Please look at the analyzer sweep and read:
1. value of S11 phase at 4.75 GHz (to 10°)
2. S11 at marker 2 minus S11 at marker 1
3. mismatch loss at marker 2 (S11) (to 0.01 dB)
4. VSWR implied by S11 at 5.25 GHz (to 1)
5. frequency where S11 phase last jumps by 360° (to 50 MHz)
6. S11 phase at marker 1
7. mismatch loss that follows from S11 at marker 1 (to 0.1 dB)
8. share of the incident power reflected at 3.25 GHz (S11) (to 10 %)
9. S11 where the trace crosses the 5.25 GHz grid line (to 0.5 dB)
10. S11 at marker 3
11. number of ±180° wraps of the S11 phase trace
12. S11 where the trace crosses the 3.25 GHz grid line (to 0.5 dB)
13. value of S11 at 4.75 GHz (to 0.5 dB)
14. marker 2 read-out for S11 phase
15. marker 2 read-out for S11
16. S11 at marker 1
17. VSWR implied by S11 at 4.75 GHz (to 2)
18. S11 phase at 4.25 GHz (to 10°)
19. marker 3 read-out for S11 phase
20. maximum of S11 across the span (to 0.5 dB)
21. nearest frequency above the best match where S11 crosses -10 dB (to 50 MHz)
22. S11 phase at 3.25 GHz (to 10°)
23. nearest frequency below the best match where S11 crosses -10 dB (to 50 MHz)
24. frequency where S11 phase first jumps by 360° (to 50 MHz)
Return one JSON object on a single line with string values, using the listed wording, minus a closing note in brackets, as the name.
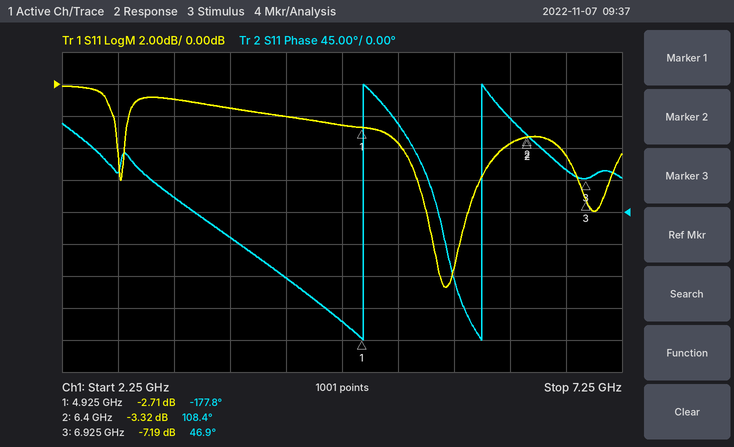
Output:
{"value of S11 phase at 4.75 GHz": "-150°", "S11 at marker 2 minus S11 at marker 1": "-0.61 dB", "mismatch loss at marker 2 (S11)": "2.72 dB", "VSWR implied by S11 at 5.25 GHz": "5", "frequency where S11 phase last jumps by 360°": "6.00 GHz", "S11 phase at marker 1": "-177.8°", "mismatch loss that follows from S11 at marker 1": "3.3 dB", "share of the incident power reflected at 3.25 GHz (S11)": "80 %", "S11 where the trace crosses the 5.25 GHz grid line": "-3.5 dB", "S11 at marker 3": "-7.19 dB", "number of ±180° wraps of the S11 phase trace": "2", "S11 where the trace crosses the 3.25 GHz grid line": "-1.0 dB", "value of S11 at 4.75 GHz": "-2.5 dB", "marker 2 read-out for S11 phase": "108.4°", "marker 2 read-out for S11": "-3.32 dB", "S11 at marker 1": "-2.71 dB", "VSWR implied by S11 at 4.75 GHz": "6", "S11 phase at 4.25 GHz": "-90°", "marker 3 read-out for S11 phase": "46.9°", "maximum of S11 across the span": "0.0 dB", "nearest frequency above the best match where S11 crosses -10 dB": "5.80 GHz", "S11 phase at 3.25 GHz": "20°", "nearest frequency below the best match where S11 crosses -10 dB": "5.55 GHz", "frequency where S11 phase first jumps by 360°": "4.95 GHz"}
